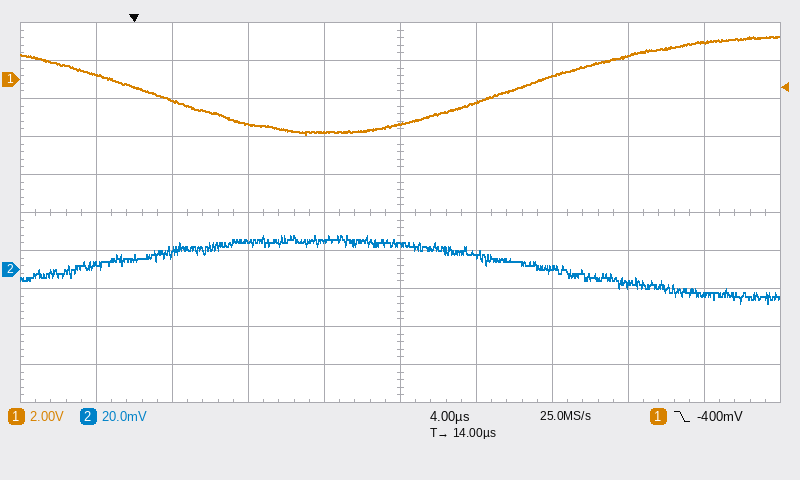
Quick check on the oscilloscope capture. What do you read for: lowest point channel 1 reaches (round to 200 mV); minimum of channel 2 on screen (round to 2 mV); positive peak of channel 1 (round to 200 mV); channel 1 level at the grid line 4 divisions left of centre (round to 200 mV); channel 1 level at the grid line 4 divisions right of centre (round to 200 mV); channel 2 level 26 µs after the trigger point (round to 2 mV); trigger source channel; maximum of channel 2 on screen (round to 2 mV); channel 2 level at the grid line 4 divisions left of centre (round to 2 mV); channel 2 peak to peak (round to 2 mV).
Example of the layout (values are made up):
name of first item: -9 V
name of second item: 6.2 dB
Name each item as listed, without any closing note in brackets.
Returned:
lowest point channel 1 reaches: -2.8 V
minimum of channel 2 on screen: -18 mV
positive peak of channel 1: 2.2 V
channel 1 level at the grid line 4 divisions left of centre: 200 mV
channel 1 level at the grid line 4 divisions right of centre: 2.0 V
channel 2 level 26 µs after the trigger point: -8 mV
trigger source channel: channel 1
maximum of channel 2 on screen: 18 mV
channel 2 level at the grid line 4 divisions left of centre: 2 mV
channel 2 peak to peak: 36 mV
